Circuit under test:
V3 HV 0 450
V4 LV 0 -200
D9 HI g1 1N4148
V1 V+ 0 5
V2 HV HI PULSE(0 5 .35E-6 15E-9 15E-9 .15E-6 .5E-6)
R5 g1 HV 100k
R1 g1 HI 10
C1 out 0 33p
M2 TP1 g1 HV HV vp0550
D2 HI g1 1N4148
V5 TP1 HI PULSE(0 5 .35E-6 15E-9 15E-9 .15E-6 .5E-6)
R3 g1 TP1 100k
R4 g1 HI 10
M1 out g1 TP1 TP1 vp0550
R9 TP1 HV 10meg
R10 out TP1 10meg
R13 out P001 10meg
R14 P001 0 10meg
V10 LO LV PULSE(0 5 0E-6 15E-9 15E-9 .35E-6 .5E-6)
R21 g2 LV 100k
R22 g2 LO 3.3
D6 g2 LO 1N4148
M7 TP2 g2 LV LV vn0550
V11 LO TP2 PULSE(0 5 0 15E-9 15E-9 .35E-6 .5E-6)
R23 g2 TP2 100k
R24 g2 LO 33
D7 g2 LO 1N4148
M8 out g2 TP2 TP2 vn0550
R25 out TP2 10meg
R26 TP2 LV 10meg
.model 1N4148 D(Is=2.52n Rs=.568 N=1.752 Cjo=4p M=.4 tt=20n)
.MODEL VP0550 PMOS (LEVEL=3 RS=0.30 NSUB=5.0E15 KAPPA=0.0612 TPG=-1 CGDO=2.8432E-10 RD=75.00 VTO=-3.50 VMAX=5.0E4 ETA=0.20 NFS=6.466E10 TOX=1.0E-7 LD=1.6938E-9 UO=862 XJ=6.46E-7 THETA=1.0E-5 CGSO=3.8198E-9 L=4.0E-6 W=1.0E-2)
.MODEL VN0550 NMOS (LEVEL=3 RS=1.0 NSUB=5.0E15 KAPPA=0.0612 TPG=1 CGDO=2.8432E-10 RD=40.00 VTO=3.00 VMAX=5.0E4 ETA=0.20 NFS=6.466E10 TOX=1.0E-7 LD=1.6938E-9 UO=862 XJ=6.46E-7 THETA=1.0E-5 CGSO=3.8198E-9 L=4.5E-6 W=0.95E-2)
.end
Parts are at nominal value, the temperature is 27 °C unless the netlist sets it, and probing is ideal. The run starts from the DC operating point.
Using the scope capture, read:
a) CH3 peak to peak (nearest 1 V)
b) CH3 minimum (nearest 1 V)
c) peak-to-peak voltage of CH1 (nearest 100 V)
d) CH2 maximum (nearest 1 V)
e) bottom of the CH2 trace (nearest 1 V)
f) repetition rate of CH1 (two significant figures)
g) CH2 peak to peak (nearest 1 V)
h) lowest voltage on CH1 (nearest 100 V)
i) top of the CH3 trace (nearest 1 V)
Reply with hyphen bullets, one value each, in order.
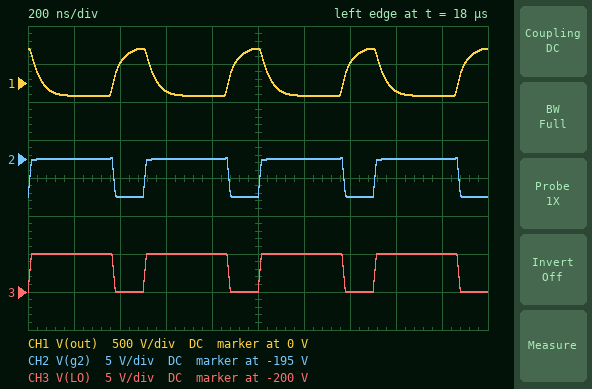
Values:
- 5 V
- -200 V
- 600 V
- -195 V
- -200 V
- 2.0 MHz
- 5 V
- -200 V
- -195 V
